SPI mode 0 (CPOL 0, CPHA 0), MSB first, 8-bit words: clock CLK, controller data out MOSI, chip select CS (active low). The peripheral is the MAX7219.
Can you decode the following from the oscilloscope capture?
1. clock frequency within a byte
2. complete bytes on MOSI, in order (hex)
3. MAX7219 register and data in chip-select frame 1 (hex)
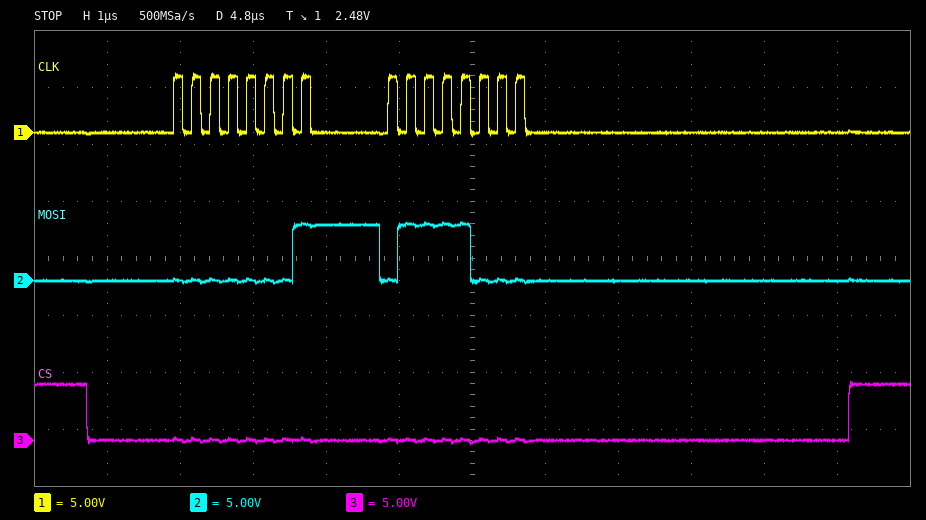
4 MHz
01 78
register 0x1, data 0x78
